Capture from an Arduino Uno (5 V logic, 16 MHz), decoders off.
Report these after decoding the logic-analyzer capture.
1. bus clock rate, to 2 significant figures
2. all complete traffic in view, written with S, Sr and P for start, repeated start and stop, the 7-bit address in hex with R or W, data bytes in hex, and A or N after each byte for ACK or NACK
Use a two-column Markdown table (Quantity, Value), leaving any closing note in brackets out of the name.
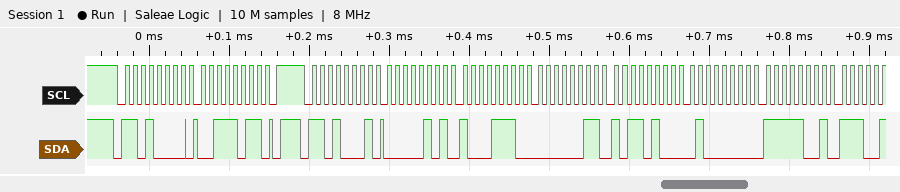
| Quantity | Value |
|---|---|
| bus clock rate, to 2 significant figures | 100 kHz |
| all complete traffic in view, written with S, Sr and P for start, repeated start and stop, the 7-bit address in hex with R or W, data bytes in hex, and A or N after each byte for ACK or NACK | S 68W A 3B A P S 68R A 05 A 8E A 03 A B4 A 40 A F9 A |
